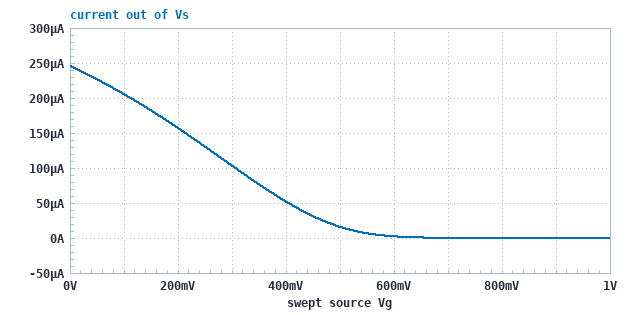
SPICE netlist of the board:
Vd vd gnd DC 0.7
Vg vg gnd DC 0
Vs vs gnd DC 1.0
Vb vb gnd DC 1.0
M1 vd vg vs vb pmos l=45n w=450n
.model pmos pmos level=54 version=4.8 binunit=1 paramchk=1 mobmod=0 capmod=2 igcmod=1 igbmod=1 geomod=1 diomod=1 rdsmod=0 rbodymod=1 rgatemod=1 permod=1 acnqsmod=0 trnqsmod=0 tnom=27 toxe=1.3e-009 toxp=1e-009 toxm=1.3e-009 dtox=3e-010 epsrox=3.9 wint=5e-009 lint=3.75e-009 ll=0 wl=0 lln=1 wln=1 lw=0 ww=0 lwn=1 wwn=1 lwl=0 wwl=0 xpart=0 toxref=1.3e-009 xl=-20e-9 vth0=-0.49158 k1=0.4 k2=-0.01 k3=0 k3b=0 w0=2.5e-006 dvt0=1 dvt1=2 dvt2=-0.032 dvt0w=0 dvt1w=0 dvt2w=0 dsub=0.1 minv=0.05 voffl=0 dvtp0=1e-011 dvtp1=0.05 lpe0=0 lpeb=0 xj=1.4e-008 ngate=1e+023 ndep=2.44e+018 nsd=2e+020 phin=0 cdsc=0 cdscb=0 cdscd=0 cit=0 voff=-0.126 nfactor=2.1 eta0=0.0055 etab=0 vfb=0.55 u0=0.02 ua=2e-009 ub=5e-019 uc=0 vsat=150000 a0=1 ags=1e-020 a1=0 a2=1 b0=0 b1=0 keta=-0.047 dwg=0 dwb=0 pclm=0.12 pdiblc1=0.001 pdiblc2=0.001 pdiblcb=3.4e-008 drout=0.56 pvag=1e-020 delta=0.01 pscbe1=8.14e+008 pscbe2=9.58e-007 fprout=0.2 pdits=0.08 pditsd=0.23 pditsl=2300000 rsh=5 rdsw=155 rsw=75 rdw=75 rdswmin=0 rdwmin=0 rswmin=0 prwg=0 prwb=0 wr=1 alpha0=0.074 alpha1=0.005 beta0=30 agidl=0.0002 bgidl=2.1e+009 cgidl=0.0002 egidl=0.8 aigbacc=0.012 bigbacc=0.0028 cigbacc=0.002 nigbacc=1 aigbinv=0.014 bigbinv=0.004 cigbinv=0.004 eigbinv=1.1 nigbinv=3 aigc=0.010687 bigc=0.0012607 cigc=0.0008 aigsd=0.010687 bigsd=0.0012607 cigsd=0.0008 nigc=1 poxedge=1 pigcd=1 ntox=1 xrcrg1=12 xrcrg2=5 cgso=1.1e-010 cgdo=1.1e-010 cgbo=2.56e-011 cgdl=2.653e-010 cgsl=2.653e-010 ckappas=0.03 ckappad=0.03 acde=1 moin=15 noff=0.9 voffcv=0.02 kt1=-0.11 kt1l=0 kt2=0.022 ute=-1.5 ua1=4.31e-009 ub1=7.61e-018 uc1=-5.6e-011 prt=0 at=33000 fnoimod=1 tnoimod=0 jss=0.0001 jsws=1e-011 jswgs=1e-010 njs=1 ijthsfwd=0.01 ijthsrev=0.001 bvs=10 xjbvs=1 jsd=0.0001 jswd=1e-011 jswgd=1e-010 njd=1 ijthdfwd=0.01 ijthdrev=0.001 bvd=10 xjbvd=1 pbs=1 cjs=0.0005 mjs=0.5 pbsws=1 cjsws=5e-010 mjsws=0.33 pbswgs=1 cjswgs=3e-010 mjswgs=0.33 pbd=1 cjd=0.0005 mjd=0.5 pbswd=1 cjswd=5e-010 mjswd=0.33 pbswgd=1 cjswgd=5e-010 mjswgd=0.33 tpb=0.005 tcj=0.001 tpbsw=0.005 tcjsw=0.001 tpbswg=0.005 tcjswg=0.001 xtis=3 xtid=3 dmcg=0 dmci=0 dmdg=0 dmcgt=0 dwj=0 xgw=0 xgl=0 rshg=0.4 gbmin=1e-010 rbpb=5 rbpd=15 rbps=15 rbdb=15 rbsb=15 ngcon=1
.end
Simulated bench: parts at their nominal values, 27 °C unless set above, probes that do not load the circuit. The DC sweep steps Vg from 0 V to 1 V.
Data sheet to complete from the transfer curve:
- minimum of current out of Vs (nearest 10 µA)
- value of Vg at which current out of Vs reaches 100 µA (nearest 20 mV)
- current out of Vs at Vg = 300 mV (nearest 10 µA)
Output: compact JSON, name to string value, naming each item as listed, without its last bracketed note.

{"minimum of current out of Vs": "0 A", "value of Vg at which current out of Vs reaches 100 µA": "300 mV", "current out of Vs at Vg = 300 mV": "100 µA"}
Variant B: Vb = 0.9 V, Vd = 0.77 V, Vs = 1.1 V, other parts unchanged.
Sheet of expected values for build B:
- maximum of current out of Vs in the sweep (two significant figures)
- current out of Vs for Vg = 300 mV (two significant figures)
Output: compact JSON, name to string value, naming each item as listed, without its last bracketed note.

{"maximum of current out of Vs in the sweep": "320 µA", "current out of Vs for Vg = 300 mV": "190 µA"}
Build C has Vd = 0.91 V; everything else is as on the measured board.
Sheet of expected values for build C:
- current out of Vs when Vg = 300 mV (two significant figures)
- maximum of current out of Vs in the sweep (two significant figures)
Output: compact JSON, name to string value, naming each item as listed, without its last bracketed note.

{"current out of Vs when Vg = 300 mV": "48 µA", "maximum of current out of Vs in the sweep": "91 µA"}
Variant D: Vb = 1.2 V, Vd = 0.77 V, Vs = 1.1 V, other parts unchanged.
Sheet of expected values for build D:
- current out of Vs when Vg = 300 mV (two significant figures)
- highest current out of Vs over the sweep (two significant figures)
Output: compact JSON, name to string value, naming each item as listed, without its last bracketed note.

{"current out of Vs when Vg = 300 mV": "150 µA", "highest current out of Vs over the sweep": "290 µA"}
